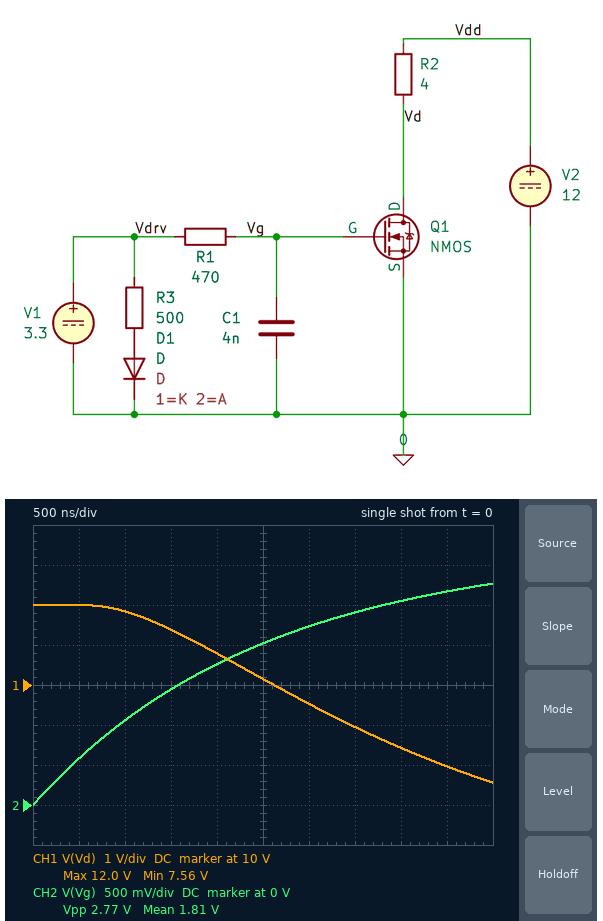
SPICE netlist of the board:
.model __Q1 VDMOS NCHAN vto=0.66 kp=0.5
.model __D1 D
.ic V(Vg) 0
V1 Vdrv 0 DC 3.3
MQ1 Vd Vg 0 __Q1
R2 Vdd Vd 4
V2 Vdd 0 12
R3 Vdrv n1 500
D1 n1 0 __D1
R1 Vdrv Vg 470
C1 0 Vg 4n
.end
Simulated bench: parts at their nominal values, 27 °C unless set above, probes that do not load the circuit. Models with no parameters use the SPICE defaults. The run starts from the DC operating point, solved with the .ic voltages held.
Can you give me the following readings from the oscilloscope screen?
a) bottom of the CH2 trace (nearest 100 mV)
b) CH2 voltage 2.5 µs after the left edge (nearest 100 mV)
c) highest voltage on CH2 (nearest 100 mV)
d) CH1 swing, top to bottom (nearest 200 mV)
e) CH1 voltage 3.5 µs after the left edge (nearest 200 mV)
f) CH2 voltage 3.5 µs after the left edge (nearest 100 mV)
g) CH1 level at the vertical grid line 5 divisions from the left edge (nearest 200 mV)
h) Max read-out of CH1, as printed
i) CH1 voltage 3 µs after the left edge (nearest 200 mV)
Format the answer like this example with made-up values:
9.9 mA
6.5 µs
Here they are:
0 V
2.0 V
2.8 V
4.4 V
9.0 V
2.4 V
10.2 V
12.0 V
9.6 V
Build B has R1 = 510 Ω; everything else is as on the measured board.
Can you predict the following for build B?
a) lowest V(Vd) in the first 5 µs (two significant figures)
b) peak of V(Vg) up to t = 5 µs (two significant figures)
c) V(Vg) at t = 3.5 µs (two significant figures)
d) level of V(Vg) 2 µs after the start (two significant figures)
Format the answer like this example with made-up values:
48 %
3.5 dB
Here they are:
7.9 V
2.7 V
2.3 V
1.7 V
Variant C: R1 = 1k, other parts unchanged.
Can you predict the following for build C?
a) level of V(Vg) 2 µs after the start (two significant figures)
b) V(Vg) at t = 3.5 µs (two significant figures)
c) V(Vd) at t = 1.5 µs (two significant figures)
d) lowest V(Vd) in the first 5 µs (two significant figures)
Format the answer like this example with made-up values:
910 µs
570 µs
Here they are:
1.0 V
1.5 V
12 V
10 V
